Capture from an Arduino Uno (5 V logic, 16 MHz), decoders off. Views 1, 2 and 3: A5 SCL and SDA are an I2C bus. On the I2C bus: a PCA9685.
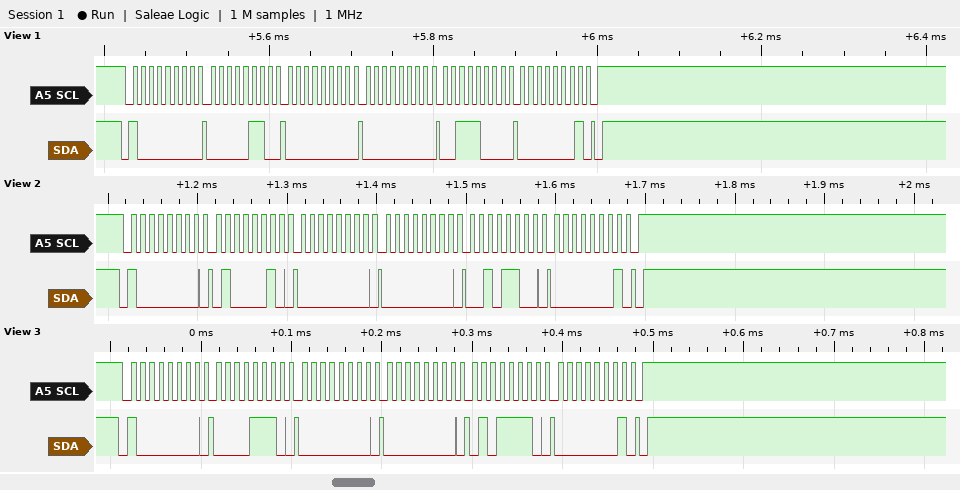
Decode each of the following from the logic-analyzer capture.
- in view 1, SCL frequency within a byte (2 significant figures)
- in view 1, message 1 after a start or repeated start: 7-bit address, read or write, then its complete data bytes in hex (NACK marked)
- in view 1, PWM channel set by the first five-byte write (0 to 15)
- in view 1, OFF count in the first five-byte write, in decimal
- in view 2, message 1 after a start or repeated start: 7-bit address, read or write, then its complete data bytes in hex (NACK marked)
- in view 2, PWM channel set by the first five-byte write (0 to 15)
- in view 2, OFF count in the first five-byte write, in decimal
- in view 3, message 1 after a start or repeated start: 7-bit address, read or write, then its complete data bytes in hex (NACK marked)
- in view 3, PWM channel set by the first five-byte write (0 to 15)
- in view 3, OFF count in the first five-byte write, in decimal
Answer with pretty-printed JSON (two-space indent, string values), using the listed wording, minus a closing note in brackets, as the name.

{
  "in view 1, SCL frequency within a byte": "100 kHz",
  "in view 1, message 1 after a start or repeated start: 7-bit address, read or write, then its complete data bytes in hex": "0x40 write: 06 00 00 38 01",
  "in view 1, PWM channel set by the first five-byte write": "0",
  "in view 1, OFF count in the first five-byte write, in decimal": "312",
  "in view 2, message 1 after a start or repeated start: 7-bit address, read or write, then its complete data bytes in hex": "0x40 write: 42 00 00 2C 01",
  "in view 2, PWM channel set by the first five-byte write": "15",
  "in view 2, OFF count in the first five-byte write, in decimal": "300",
  "in view 3, message 1 after a start or repeated start: 7-bit address, read or write, then its complete data bytes in hex": "0x40 write: 0E 00 00 5E 01",
  "in view 3, PWM channel set by the first five-byte write": "2",
  "in view 3, OFF count in the first five-byte write, in decimal": "350"
}
